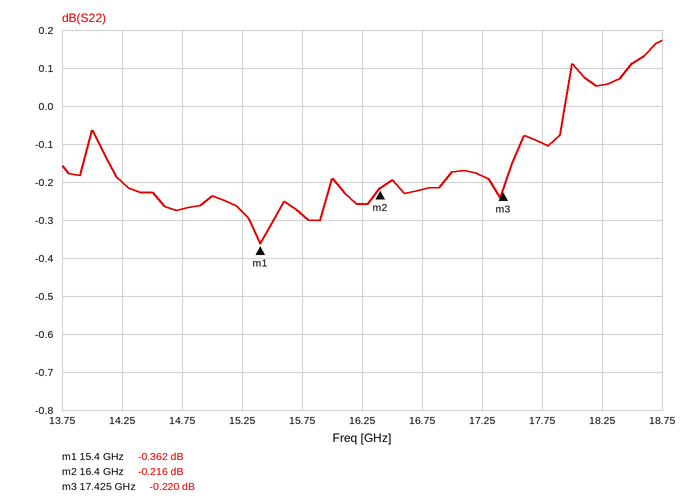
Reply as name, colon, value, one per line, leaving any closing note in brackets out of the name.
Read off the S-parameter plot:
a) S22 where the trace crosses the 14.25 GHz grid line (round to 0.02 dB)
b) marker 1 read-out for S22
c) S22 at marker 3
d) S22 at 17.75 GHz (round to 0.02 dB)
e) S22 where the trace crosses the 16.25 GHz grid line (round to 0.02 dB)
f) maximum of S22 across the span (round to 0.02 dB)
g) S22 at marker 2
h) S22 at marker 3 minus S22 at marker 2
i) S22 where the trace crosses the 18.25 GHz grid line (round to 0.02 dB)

S22 where the trace crosses the 14.25 GHz grid line: -0.20 dB
marker 1 read-out for S22: -0.362 dB
S22 at marker 3: -0.220 dB
S22 at 17.75 GHz: -0.10 dB
S22 where the trace crosses the 16.25 GHz grid line: -0.26 dB
maximum of S22 across the span: 0.18 dB
S22 at marker 2: -0.216 dB
S22 at marker 3 minus S22 at marker 2: -0.004 dB
S22 where the trace crosses the 18.25 GHz grid line: 0.06 dB
